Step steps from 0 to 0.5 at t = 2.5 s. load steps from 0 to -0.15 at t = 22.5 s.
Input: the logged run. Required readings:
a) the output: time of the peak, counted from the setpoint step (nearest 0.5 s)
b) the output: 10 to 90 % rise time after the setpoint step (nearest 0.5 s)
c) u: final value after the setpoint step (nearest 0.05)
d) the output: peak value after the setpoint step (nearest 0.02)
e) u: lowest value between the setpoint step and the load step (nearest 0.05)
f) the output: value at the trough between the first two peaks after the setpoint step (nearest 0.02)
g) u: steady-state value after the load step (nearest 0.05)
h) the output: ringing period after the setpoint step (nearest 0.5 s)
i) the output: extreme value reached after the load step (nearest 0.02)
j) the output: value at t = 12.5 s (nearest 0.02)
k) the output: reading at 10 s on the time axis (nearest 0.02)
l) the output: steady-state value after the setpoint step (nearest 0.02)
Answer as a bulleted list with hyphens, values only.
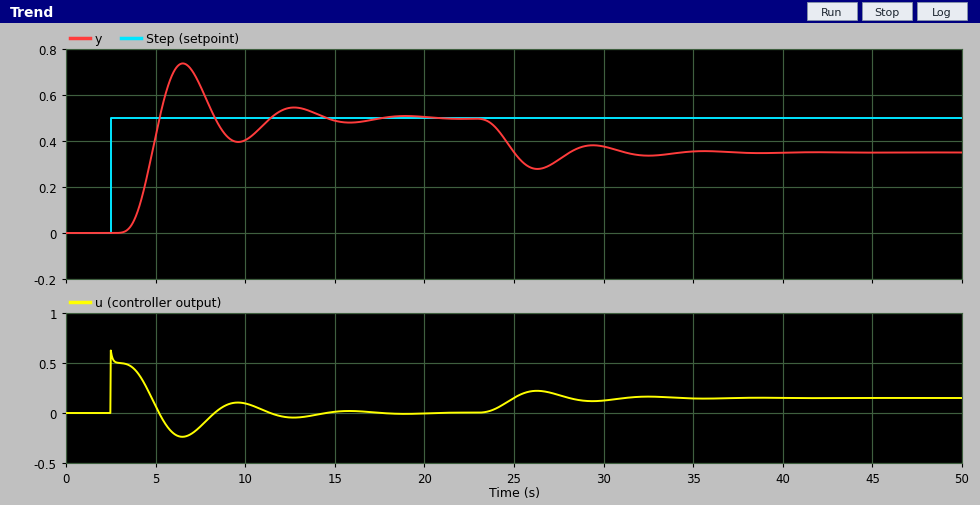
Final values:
- 4.0 s
- 1.5 s
- 0.00
- 0.74
- -0.25
- 0.40
- 0.15
- 6.0 s
- 0.28
- 0.54
- 0.40
- 0.50
